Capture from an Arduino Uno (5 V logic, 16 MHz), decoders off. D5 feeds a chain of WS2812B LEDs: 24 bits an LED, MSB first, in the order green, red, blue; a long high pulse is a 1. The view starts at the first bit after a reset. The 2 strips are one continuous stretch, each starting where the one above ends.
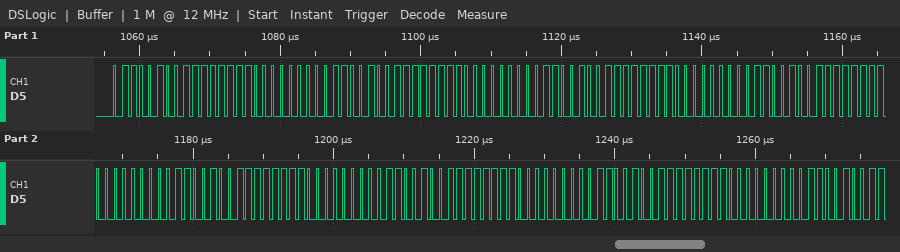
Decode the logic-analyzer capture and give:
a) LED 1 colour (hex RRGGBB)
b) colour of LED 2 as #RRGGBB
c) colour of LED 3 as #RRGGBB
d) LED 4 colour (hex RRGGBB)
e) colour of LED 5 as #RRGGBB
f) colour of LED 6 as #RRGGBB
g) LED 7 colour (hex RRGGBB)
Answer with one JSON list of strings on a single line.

["#FF6400", "#FF6400", "#FF6400", "#FF6400", "#FF6400", "#FF6400", "#FF6400"]
